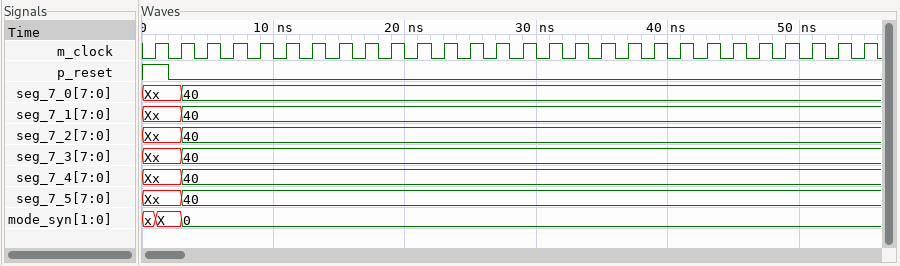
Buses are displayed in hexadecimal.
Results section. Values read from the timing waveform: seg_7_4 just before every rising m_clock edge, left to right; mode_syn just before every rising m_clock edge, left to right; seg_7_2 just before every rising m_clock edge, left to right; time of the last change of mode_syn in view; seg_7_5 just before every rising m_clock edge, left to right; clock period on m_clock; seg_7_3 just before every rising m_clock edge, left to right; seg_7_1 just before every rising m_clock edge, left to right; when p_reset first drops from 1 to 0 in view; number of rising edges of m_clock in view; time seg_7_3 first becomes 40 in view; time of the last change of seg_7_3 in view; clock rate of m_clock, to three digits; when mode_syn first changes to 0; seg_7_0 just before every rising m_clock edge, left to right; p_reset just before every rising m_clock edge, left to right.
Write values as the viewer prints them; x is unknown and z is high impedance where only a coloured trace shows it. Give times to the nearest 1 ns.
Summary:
Xx, Xx, 40, 40, 40, 40, 40, 40, 40, 40, 40, 40, 40, 40, 40, 40, 40, 40, 40, 40, 40, 40, 40, 40, 40, 40, 40, 40
x, X, 0, 0, 0, 0, 0, 0, 0, 0, 0, 0, 0, 0, 0, 0, 0, 0, 0, 0, 0, 0, 0, 0, 0, 0, 0, 0
Xx, Xx, 40, 40, 40, 40, 40, 40, 40, 40, 40, 40, 40, 40, 40, 40, 40, 40, 40, 40, 40, 40, 40, 40, 40, 40, 40, 40
3 ns
Xx, Xx, 40, 40, 40, 40, 40, 40, 40, 40, 40, 40, 40, 40, 40, 40, 40, 40, 40, 40, 40, 40, 40, 40, 40, 40, 40, 40
2 ns
Xx, Xx, 40, 40, 40, 40, 40, 40, 40, 40, 40, 40, 40, 40, 40, 40, 40, 40, 40, 40, 40, 40, 40, 40, 40, 40, 40, 40
Xx, Xx, 40, 40, 40, 40, 40, 40, 40, 40, 40, 40, 40, 40, 40, 40, 40, 40, 40, 40, 40, 40, 40, 40, 40, 40, 40, 40
2 ns
28
3 ns
3 ns
500 MHz
3 ns
Xx, Xx, 40, 40, 40, 40, 40, 40, 40, 40, 40, 40, 40, 40, 40, 40, 40, 40, 40, 40, 40, 40, 40, 40, 40, 40, 40, 40
1 0 0 0 0 0 0 0 0 0 0 0 0 0 0 0 0 0 0 0 0 0 0 0 0 0 0 0
